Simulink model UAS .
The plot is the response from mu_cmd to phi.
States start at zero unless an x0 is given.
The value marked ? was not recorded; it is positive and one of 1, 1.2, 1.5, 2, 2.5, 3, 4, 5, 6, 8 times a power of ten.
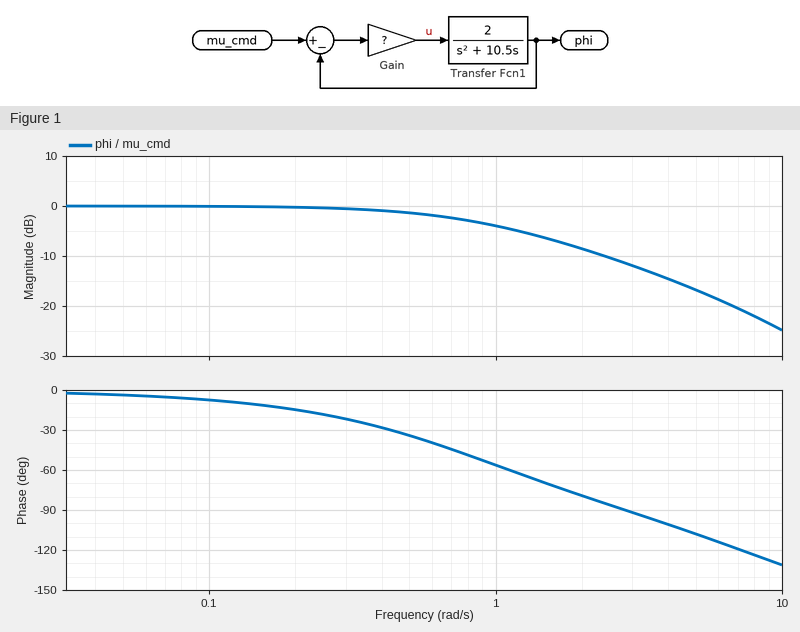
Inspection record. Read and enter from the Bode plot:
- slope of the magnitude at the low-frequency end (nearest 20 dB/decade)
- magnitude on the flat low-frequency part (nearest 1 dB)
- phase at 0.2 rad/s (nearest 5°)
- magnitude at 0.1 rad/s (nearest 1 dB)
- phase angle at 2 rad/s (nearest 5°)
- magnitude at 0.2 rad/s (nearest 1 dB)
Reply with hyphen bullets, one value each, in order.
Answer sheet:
- 0 dB/decade
- 0 dB
- -15°
- 0 dB
- -80°
- 0 dB
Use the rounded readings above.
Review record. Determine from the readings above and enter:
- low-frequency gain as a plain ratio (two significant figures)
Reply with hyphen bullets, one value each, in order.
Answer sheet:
- 1.0
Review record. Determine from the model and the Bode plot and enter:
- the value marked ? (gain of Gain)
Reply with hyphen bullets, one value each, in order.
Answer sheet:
- 4
